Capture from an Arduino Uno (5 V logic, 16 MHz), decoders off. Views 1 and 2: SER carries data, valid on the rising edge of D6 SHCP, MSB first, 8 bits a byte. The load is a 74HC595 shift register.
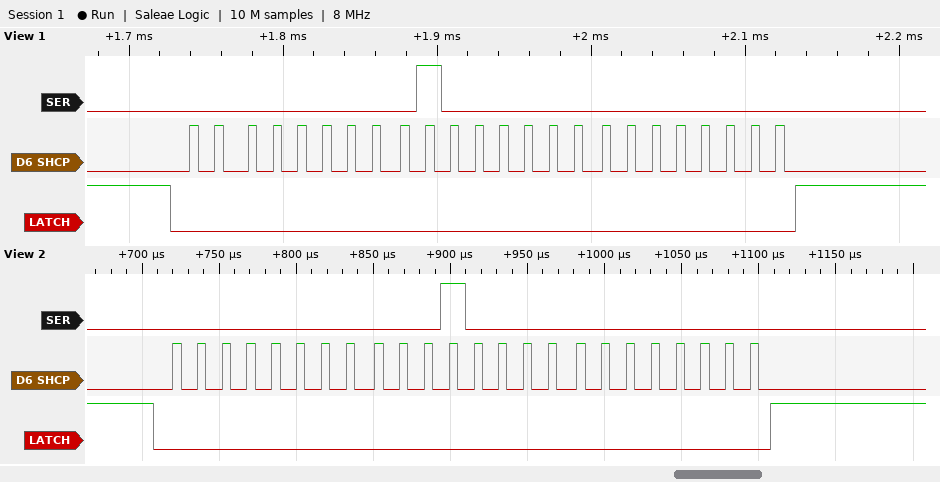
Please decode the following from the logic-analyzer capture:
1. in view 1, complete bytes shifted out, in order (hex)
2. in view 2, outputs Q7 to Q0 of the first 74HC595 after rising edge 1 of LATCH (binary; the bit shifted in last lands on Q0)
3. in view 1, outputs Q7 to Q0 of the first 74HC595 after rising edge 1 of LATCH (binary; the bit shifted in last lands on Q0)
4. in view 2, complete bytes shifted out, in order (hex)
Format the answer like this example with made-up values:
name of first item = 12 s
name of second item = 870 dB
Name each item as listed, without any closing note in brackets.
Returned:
in view 1, complete bytes shifted out, in order = 00 40 00
in view 2, outputs Q7 to Q0 of the first 74HC595 after rising edge 1 of LATCH = 00000000
in view 1, outputs Q7 to Q0 of the first 74HC595 after rising edge 1 of LATCH = 00000000
in view 2, complete bytes shifted out, in order = 0x00 0x10 0x00
